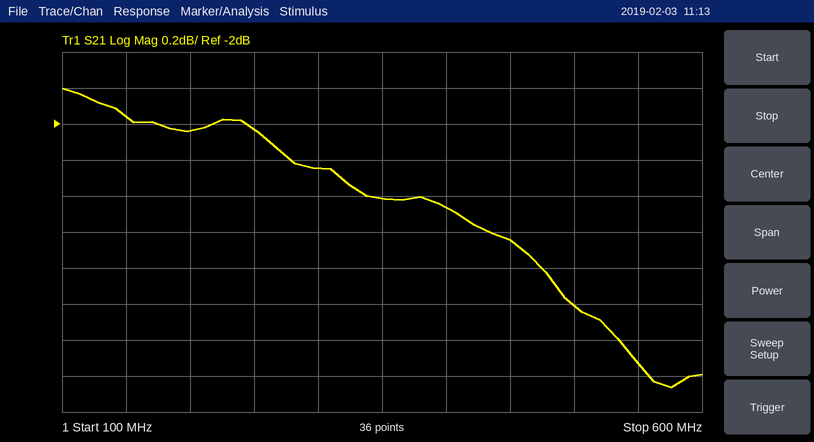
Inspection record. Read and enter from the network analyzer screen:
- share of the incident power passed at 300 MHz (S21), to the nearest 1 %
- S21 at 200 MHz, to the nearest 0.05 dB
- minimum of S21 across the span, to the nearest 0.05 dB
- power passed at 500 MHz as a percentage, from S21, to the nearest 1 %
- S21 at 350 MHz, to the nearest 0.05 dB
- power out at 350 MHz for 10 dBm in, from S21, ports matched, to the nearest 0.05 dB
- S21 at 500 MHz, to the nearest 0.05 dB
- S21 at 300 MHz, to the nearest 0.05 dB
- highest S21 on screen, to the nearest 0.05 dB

60 %
-2.05 dB
-3.45 dB
50 %
-2.40 dB
7.60 dBm
-3.00 dB
-2.25 dB
-1.80 dB
